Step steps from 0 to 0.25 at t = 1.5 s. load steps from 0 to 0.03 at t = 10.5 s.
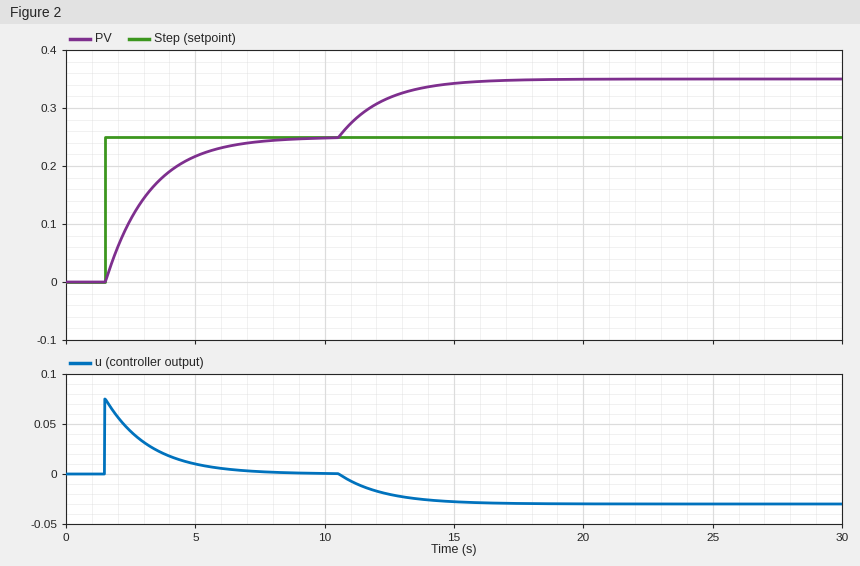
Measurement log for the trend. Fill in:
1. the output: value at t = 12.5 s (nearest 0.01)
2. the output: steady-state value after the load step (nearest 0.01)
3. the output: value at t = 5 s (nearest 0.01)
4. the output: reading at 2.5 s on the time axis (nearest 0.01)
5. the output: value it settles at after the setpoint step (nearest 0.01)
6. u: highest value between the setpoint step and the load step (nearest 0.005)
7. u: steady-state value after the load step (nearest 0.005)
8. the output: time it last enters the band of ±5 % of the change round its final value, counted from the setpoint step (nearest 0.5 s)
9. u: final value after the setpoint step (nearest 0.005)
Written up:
0.32
0.35
0.22
0.11
0.25
0.075
-0.030
5.0 s
0.000
